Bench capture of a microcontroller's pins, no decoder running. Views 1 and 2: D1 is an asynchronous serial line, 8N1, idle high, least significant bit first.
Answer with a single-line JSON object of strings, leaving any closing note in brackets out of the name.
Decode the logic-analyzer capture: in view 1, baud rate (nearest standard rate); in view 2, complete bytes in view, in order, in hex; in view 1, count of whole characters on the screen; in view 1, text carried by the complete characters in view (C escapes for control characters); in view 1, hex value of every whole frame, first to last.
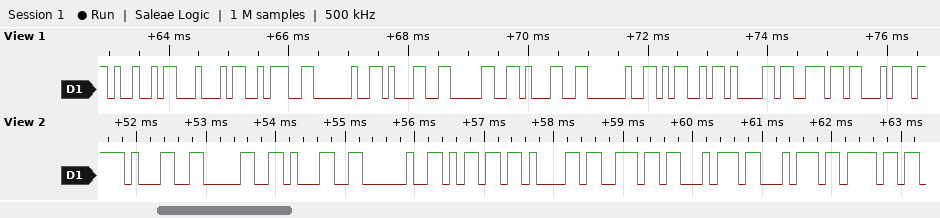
{"in view 1, baud rate": "9600 baud", "in view 2, complete bytes in view, in order, in hex": "31 30 31 20 6D 61 6E 74 74 6F", "in view 1, count of whole characters on the screen": "12", "in view 1, text carried by the complete characters in view": "\"ID: 101 Mant\"", "in view 1, hex value of every whole frame, first to last": "49 44 3A 20 31 30 31 20 4D 61 6E 74"}
